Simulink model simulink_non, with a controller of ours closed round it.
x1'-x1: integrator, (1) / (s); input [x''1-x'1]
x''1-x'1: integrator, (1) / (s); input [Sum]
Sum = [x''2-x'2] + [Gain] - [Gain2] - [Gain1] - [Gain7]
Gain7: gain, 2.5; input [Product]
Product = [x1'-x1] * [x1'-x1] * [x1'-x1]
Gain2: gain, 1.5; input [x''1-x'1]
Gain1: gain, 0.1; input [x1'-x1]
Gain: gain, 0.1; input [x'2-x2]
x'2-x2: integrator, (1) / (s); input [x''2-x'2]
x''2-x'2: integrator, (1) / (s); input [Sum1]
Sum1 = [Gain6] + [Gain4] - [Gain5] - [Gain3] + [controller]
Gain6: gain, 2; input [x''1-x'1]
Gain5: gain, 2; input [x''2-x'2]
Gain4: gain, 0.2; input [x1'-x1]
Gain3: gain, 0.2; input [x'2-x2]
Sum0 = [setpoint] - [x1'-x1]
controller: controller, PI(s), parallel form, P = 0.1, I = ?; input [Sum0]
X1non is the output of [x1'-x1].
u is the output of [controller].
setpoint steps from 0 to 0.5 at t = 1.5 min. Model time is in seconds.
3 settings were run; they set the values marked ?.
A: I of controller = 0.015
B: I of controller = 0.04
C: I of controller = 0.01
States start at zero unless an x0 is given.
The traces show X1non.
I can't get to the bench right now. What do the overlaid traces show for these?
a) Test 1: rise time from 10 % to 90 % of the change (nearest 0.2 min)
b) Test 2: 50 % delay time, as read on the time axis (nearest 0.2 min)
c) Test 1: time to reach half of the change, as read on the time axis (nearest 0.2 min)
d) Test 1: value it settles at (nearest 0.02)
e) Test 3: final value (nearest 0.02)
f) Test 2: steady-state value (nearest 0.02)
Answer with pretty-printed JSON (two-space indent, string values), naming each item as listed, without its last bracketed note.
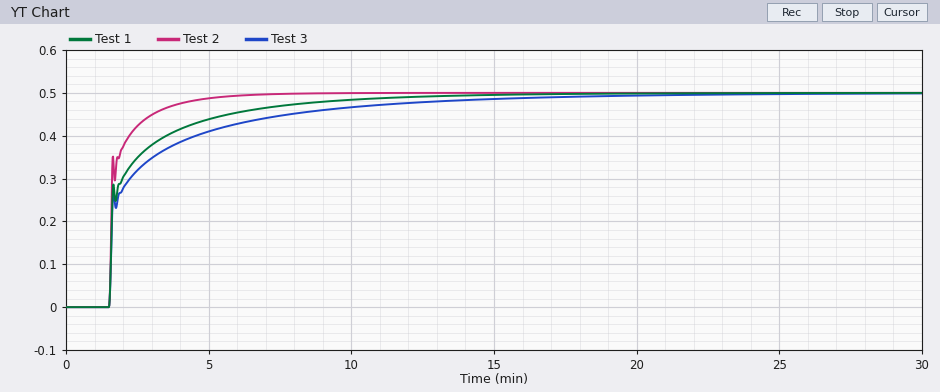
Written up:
{
  "Test 1: rise time from 10 % to 90 % of the change": "4.2 min",
  "Test 2: 50 % delay time, as read on the time axis": "1.6 min",
  "Test 1: time to reach half of the change, as read on the time axis": "1.6 min",
  "Test 1: value it settles at": "0.50",
  "Test 3: final value": "0.50",
  "Test 2: steady-state value": "0.50"
}
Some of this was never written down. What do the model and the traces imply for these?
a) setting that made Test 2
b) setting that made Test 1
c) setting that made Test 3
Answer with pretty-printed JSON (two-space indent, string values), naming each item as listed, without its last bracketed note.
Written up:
{
  "setting that made Test 2": "B",
  "setting that made Test 1": "A",
  "setting that made Test 3": "C"
}
